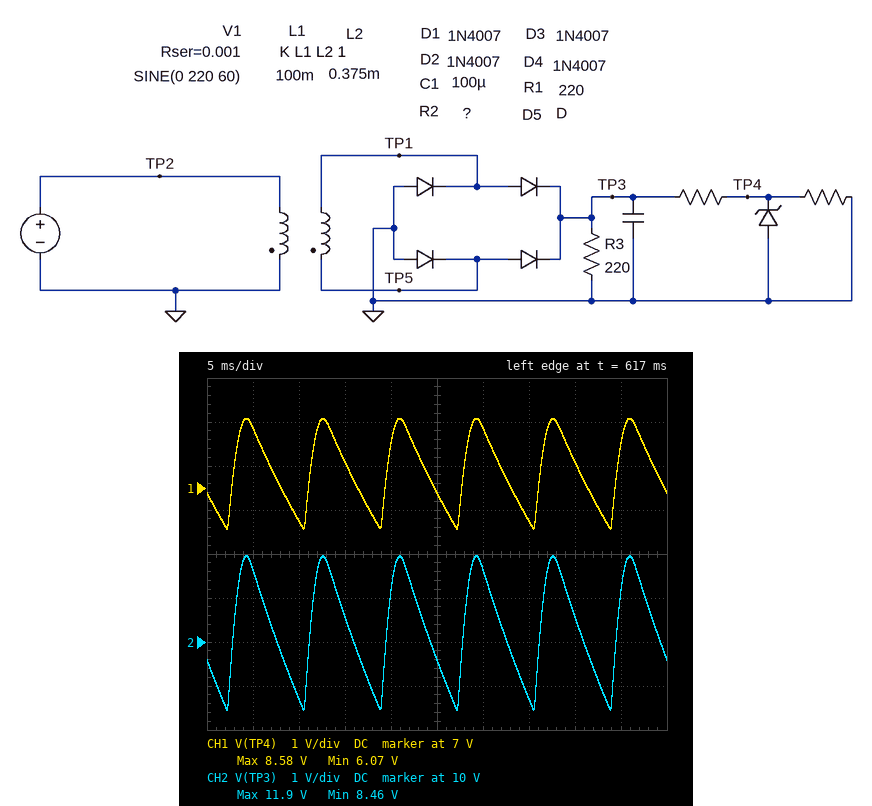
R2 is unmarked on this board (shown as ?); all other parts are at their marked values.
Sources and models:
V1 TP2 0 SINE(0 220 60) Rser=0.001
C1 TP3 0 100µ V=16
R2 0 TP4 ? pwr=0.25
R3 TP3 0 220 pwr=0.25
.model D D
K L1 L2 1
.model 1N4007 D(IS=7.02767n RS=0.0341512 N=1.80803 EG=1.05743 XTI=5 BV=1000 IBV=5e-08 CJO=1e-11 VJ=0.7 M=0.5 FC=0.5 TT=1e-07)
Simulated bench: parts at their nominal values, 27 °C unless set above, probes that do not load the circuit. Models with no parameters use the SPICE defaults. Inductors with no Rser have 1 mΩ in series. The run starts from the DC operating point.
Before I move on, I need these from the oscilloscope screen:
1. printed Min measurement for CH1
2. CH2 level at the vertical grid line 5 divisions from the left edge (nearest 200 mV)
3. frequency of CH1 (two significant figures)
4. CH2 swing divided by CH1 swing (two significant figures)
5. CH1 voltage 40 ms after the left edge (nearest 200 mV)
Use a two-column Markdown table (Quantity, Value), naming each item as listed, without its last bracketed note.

| Quantity | Value |
|---|---|
| printed Min measurement for CH1 | 6.07 V |
| CH2 level at the vertical grid line 5 divisions from the left edge | 9.6 V |
| frequency of CH1 | 120 Hz |
| CH2 swing divided by CH1 swing | 1.4 |
| CH1 voltage 40 ms after the left edge | 7.6 V |
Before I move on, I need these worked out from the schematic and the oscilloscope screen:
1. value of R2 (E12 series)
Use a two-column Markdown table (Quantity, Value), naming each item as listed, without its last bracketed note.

| Quantity | Value |
|---|---|
| value of R2 | 560 Ω |
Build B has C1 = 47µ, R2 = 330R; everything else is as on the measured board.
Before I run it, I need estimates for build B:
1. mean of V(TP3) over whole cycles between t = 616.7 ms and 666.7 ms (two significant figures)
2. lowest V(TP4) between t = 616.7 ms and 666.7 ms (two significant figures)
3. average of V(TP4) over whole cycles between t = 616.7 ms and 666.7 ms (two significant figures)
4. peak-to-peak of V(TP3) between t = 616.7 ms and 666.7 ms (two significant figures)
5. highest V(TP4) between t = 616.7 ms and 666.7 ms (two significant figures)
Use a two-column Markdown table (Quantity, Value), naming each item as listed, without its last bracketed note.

| Quantity | Value |
|---|---|
| mean of V(TP3) over whole cycles between t = 616.7 ms and 666.7 ms | 9.2 V |
| lowest V(TP4) between t = 616.7 ms and 666.7 ms | 3.6 V |
| average of V(TP4) over whole cycles between t = 616.7 ms and 666.7 ms | 5.5 V |
| peak-to-peak of V(TP3) between t = 616.7 ms and 666.7 ms | 6.0 V |
| highest V(TP4) between t = 616.7 ms and 666.7 ms | 7.2 V |
